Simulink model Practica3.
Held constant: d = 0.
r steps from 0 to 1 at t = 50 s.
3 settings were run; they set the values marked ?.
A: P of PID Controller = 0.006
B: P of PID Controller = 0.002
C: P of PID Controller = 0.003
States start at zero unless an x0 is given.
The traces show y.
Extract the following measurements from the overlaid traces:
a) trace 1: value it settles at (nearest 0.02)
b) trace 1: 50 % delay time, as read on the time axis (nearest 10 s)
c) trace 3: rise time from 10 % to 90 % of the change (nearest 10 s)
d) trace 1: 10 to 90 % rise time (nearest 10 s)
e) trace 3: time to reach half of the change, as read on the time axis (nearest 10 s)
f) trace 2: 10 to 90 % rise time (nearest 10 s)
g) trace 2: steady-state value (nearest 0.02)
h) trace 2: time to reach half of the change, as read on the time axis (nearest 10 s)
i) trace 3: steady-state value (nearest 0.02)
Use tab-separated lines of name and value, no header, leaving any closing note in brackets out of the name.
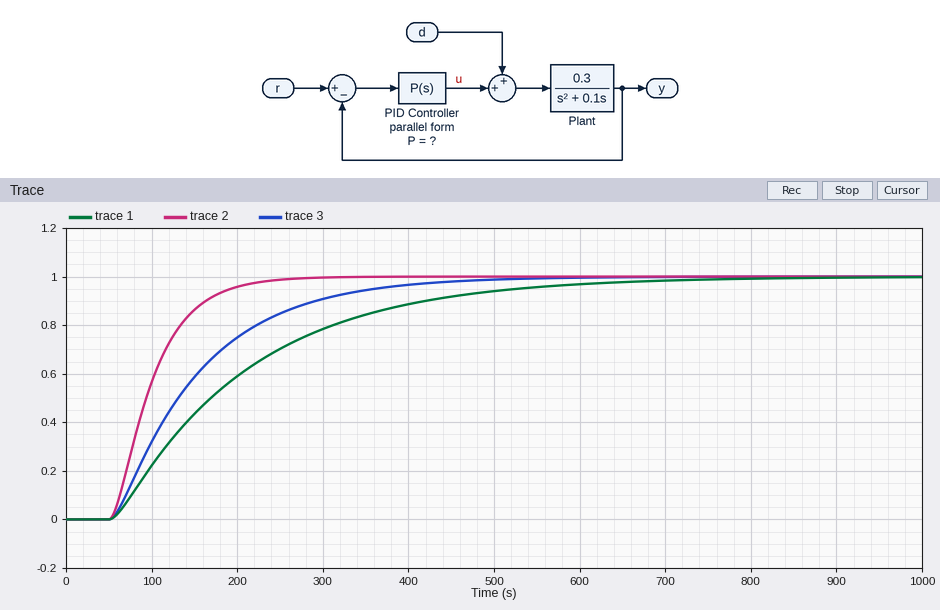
trace 1: value it settles at	1.00
trace 1: 50 % delay time, as read on the time axis	170 s
trace 3: rise time from 10 % to 90 % of the change	220 s
trace 1: 10 to 90 % rise time	340 s
trace 3: time to reach half of the change, as read on the time axis	130 s
trace 2: 10 to 90 % rise time	100 s
trace 2: steady-state value	1.00
trace 2: time to reach half of the change, as read on the time axis	90 s
trace 3: steady-state value	1.00
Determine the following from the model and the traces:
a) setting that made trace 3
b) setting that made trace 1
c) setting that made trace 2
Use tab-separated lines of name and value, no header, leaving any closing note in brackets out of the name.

setting that made trace 3	C
setting that made trace 1	B
setting that made trace 2	A
